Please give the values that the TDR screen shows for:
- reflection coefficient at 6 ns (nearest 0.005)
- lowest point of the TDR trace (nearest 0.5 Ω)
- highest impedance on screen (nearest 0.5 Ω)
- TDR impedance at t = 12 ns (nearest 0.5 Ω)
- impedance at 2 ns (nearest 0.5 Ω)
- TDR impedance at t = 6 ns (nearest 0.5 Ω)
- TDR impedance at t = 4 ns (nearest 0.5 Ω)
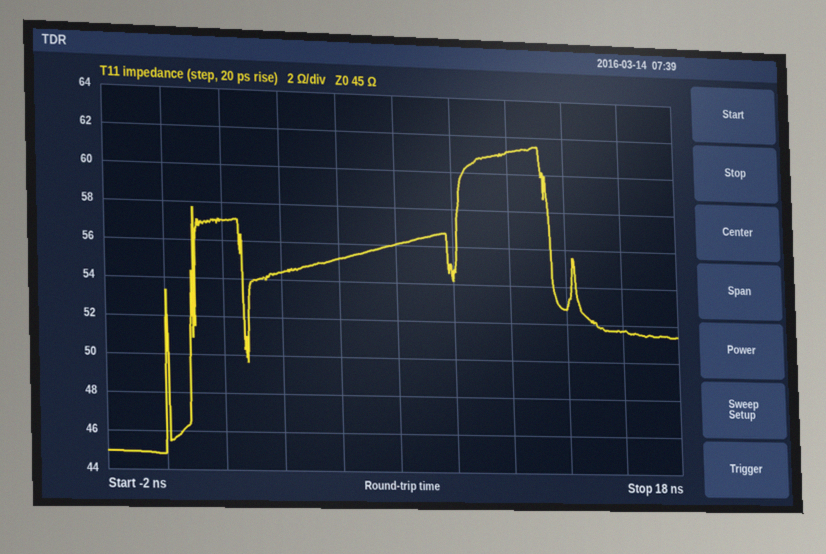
+0.100
45.0 Ω
61.5 Ω
61.0 Ω
57.0 Ω
55.0 Ω
54.5 Ω
